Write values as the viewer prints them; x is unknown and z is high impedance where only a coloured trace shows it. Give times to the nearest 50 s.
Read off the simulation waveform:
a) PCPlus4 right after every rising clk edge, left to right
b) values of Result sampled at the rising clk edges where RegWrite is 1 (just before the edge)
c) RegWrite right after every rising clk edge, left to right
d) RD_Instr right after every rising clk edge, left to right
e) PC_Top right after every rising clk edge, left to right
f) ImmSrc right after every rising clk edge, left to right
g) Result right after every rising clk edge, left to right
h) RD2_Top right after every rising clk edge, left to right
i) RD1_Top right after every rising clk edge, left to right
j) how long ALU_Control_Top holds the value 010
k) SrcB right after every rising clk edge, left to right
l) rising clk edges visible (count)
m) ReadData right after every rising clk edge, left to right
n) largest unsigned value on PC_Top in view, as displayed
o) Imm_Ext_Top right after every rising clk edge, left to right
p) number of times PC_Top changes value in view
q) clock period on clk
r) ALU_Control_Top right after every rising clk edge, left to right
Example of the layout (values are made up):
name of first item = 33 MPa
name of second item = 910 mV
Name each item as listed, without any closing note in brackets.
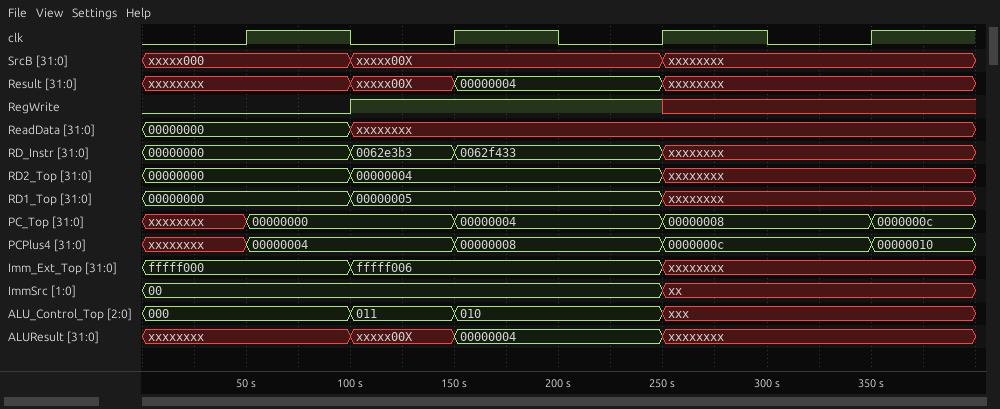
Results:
PCPlus4 right after every rising clk edge, left to right = 00000004, 00000008, 0000000c, 00000010
values of Result sampled at the rising clk edges where RegWrite is 1 = xxxxx00X, 00000004
RegWrite right after every rising clk edge, left to right = 0 1 x x
RD_Instr right after every rising clk edge, left to right = 00000000, 0062f433, xxxxxxxx, xxxxxxxx
PC_Top right after every rising clk edge, left to right = 00000000, 00000004, 00000008, 0000000c
ImmSrc right after every rising clk edge, left to right = 00, 00, xx, xx
Result right after every rising clk edge, left to right = xxxxxxxx, 00000004, xxxxxxxx, xxxxxxxx
RD2_Top right after every rising clk edge, left to right = 00000000, 00000004, xxxxxxxx, xxxxxxxx
RD1_Top right after every rising clk edge, left to right = 00000000, 00000005, xxxxxxxx, xxxxxxxx
how long ALU_Control_Top holds the value 010 = 100 s
SrcB right after every rising clk edge, left to right = xxxxx000, xxxxx00X, xxxxxxxx, xxxxxxxx
rising clk edges visible = 4
ReadData right after every rising clk edge, left to right = 00000000, xxxxxxxx, xxxxxxxx, xxxxxxxx
largest unsigned value on PC_Top in view, as displayed = 0000000c
Imm_Ext_Top right after every rising clk edge, left to right = fffff000, fffff006, xxxxxxxx, xxxxxxxx
number of times PC_Top changes value in view = 4
clock period on clk = 100 s
ALU_Control_Top right after every rising clk edge, left to right = 000, 010, xxx, xxx
